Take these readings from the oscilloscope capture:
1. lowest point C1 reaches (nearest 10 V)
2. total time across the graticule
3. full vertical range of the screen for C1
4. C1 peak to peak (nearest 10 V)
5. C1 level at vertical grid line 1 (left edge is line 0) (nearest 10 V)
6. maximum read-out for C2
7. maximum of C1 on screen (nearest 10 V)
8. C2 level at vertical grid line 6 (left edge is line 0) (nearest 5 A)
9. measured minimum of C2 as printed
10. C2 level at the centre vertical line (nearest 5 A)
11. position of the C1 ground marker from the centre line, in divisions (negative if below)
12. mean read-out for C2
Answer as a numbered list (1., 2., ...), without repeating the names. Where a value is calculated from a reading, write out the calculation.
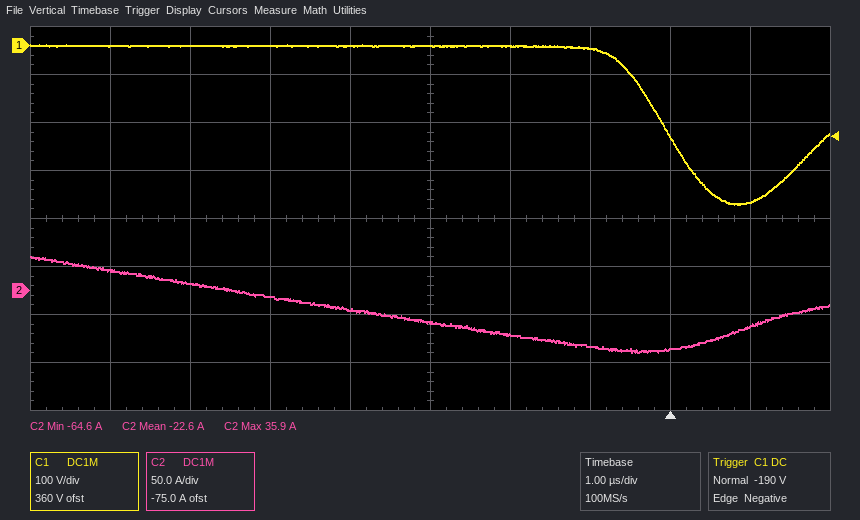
1. -330 V
2. 10 µs
3. 800 V
4. 0 V − (-330 V) = 330 V
5. 0 V
6. 35.9 A
7. 0 V
8. -45 A
9. -64.6 A
10. -35 A
11. +3.6 div
12. -22.6 A
